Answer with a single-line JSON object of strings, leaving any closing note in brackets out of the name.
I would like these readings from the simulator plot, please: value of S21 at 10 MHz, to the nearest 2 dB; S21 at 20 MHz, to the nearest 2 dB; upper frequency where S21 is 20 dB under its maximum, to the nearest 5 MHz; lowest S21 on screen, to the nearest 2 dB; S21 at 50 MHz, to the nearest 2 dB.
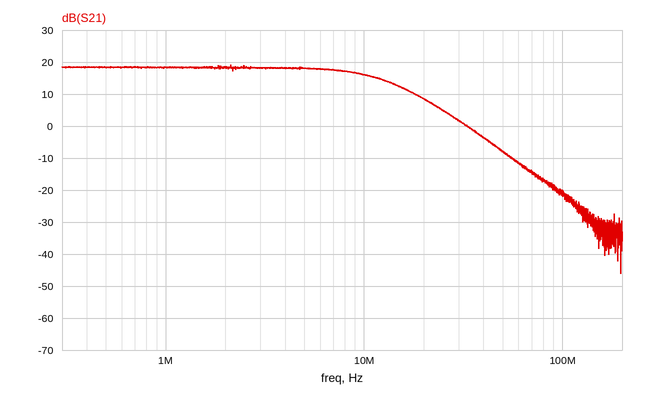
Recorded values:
{"value of S21 at 10 MHz, to the nearest 2 dB": "16 dB", "S21 at 20 MHz, to the nearest 2 dB": "8 dB", "upper frequency where S21 is 20 dB under its maximum, to the nearest 5 MHz": "35 MHz", "lowest S21 on screen, to the nearest 2 dB": "-46 dB", "S21 at 50 MHz, to the nearest 2 dB": "-8 dB"}
